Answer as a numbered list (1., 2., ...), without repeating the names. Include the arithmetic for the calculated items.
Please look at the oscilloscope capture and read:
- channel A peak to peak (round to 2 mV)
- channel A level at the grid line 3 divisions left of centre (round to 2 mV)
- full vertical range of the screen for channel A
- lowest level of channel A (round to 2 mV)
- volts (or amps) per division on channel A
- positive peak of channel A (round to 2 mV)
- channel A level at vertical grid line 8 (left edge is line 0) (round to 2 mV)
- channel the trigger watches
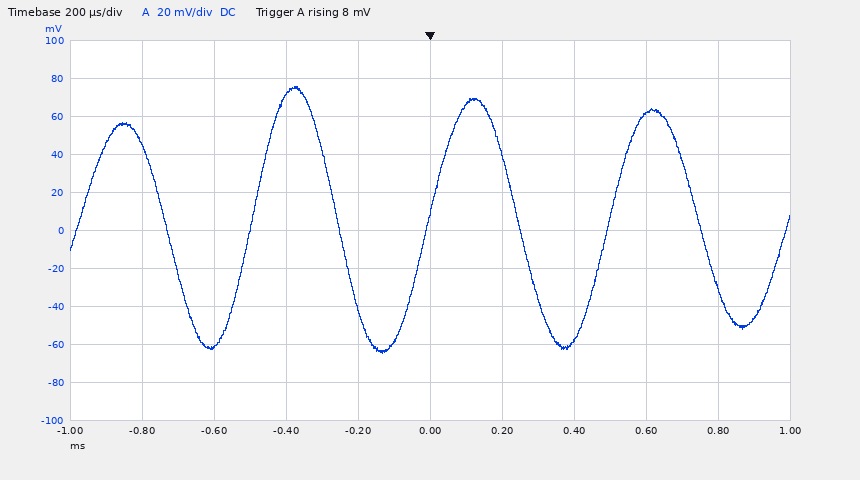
1. 76 mV − (-64 mV) = 140 mV
2. -62 mV
3. 200 mV
4. -64 mV
5. 20 mV
6. 76 mV
7. 62 mV
8. channel A
